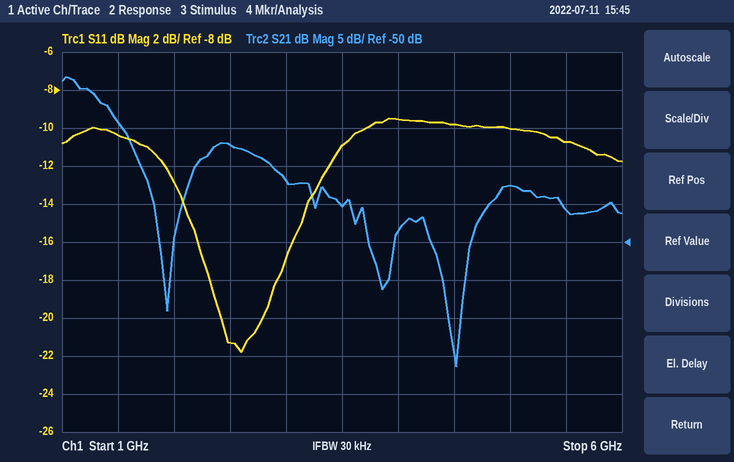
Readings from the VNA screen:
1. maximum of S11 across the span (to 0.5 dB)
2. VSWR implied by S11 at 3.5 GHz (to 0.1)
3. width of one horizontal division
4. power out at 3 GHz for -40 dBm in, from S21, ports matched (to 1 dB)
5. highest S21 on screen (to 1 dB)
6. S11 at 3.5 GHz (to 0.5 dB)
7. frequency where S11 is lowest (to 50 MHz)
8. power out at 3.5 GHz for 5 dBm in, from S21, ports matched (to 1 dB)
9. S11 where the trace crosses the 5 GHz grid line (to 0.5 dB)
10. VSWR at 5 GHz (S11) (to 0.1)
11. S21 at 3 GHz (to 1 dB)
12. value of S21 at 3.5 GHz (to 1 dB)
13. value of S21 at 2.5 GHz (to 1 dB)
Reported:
-9.5 dB
1.8
500 MHz
-82 dBm
-28 dB
-11.0 dB
2.60 GHz
-40 dBm
-10.0 dB
1.9
-42 dB
-45 dB
-37 dB
